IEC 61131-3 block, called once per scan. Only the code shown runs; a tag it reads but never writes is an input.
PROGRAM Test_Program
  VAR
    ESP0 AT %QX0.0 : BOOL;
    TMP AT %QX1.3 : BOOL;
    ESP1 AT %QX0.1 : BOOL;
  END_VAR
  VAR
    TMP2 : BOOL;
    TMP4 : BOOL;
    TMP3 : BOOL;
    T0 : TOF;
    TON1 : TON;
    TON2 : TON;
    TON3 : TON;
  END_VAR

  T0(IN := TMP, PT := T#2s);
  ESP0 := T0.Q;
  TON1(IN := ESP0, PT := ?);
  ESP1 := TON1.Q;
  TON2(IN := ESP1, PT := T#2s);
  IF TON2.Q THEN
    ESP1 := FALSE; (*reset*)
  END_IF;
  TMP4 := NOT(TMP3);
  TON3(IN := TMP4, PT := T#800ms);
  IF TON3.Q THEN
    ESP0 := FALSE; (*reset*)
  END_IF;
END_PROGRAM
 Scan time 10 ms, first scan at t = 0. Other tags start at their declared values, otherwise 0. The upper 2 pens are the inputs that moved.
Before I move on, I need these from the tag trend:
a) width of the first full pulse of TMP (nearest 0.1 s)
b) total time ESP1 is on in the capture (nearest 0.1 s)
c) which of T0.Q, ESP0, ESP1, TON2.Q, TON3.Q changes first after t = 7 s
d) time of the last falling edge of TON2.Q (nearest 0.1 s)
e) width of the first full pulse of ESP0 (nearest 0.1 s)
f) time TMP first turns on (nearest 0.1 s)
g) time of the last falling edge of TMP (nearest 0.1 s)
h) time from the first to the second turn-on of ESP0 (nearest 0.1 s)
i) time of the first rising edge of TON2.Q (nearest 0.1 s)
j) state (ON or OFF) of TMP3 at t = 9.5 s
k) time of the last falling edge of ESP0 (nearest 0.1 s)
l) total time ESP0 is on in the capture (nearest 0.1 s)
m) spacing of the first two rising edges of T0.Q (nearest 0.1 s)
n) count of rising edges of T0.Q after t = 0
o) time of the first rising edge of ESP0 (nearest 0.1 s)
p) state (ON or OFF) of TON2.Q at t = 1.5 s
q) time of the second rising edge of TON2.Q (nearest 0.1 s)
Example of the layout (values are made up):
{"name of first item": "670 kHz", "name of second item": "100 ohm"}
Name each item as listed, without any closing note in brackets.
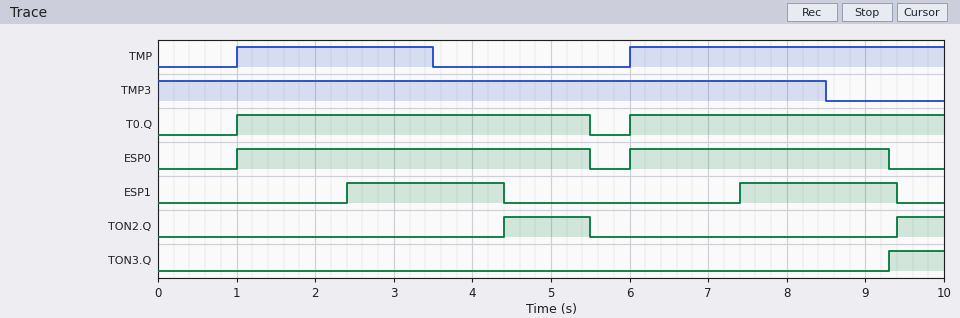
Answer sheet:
{"width of the first full pulse of TMP": "2.5 s", "total time ESP1 is on in the capture": "4.0 s", "which of T0.Q, ESP0, ESP1, TON2.Q, TON3.Q changes first after t = 7 s": "ESP1", "time of the last falling edge of TON2.Q": "5.5 s", "width of the first full pulse of ESP0": "4.5 s", "time TMP first turns on": "1.0 s", "time of the last falling edge of TMP": "3.5 s", "time from the first to the second turn-on of ESP0": "5.0 s", "time of the first rising edge of TON2.Q": "4.4 s", "state (ON or OFF) of TMP3 at t = 9.5 s": "OFF", "time of the last falling edge of ESP0": "9.3 s", "total time ESP0 is on in the capture": "7.8 s", "spacing of the first two rising edges of T0.Q": "5.0 s", "count of rising edges of T0.Q after t = 0": "2", "time of the first rising edge of ESP0": "1.0 s", "state (ON or OFF) of TON2.Q at t = 1.5 s": "OFF", "time of the second rising edge of TON2.Q": "9.4 s"}
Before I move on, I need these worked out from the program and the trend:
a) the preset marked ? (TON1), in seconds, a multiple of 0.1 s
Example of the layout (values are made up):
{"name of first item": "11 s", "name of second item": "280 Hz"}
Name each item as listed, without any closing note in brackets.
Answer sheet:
{"the preset marked ? (TON1), in seconds, a multiple of 0.1 s": "1.4 s"}
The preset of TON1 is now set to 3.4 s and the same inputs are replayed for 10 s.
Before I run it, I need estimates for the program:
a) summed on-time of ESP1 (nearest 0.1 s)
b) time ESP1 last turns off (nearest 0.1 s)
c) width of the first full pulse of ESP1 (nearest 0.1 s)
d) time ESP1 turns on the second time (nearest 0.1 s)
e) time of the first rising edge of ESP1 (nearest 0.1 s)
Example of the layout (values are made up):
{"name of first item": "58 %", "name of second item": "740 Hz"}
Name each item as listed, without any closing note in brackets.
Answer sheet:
{"summed on-time of ESP1": "1.7 s", "time ESP1 last turns off": "5.5 s", "width of the first full pulse of ESP1": "1.1 s", "time ESP1 turns on the second time": "9.4 s", "time of the first rising edge of ESP1": "4.4 s"}
